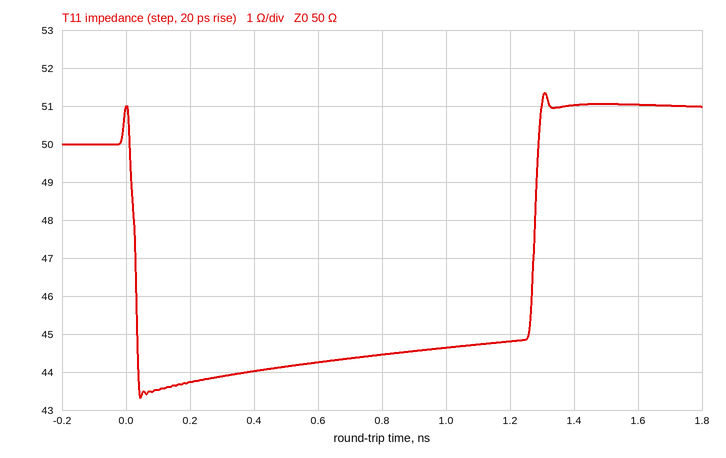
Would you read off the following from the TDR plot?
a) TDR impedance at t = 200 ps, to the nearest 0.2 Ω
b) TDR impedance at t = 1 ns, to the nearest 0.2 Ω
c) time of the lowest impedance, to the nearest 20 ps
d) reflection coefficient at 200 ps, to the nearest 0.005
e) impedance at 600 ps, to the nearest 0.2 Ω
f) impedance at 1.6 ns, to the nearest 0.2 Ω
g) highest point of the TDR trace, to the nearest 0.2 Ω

43.8 Ω
44.6 Ω
40 ps
-0.065
44.2 Ω
51.0 Ω
51.4 Ω
